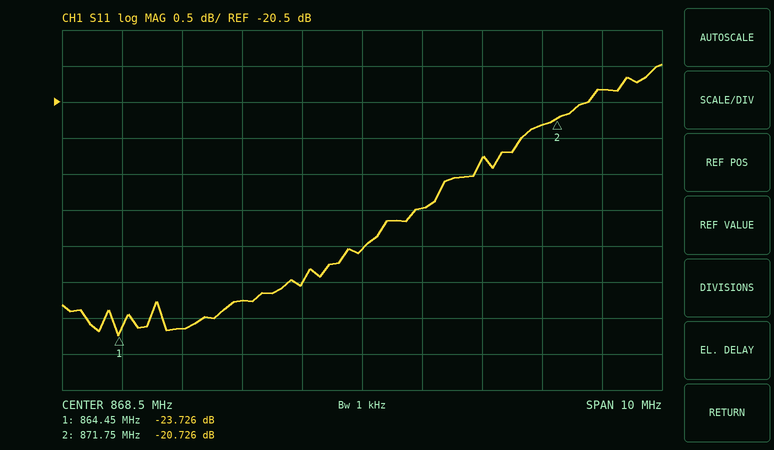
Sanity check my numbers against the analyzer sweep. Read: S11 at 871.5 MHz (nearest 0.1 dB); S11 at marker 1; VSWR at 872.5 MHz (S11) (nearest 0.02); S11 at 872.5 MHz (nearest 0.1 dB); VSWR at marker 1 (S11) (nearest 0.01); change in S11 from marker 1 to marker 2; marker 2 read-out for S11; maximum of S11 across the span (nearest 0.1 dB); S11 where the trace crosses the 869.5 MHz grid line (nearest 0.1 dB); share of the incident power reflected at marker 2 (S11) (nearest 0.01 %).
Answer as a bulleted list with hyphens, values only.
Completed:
- -20.8 dB
- -23.726 dB
- 1.22
- -20.3 dB
- 1.14
- 3.000 dB
- -20.726 dB
- -20.0 dB
- -22.0 dB
- 0.85 %
